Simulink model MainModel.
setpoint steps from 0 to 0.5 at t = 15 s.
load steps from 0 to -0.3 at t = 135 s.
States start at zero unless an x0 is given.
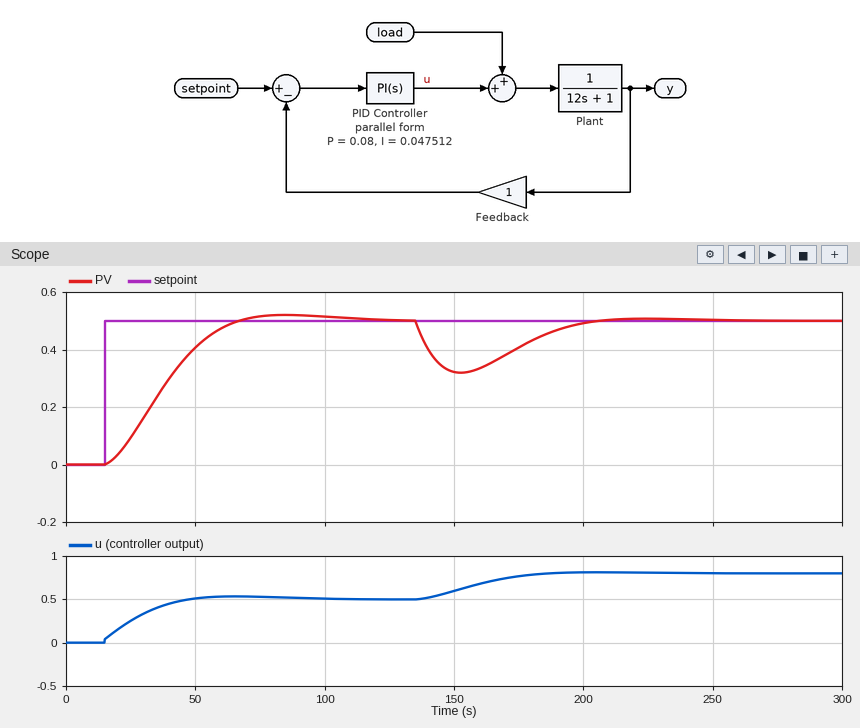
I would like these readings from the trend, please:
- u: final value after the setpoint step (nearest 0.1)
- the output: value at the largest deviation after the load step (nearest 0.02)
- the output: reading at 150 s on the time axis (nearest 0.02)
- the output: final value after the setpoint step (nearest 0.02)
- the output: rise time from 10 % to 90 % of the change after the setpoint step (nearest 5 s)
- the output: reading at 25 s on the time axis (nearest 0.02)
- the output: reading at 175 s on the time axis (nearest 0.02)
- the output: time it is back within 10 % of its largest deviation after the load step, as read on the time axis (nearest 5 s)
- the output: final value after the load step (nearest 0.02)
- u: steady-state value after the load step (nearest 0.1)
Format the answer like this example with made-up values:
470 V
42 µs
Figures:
0.5
0.32
0.32
0.50
35 s
0.10
0.40
195 s
0.50
0.8
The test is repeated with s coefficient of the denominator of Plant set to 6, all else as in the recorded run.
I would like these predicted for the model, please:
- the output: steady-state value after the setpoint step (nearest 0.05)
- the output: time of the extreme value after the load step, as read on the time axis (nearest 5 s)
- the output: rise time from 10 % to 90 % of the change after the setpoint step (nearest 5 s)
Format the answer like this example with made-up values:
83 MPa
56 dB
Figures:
0.50
145 s
40 s
